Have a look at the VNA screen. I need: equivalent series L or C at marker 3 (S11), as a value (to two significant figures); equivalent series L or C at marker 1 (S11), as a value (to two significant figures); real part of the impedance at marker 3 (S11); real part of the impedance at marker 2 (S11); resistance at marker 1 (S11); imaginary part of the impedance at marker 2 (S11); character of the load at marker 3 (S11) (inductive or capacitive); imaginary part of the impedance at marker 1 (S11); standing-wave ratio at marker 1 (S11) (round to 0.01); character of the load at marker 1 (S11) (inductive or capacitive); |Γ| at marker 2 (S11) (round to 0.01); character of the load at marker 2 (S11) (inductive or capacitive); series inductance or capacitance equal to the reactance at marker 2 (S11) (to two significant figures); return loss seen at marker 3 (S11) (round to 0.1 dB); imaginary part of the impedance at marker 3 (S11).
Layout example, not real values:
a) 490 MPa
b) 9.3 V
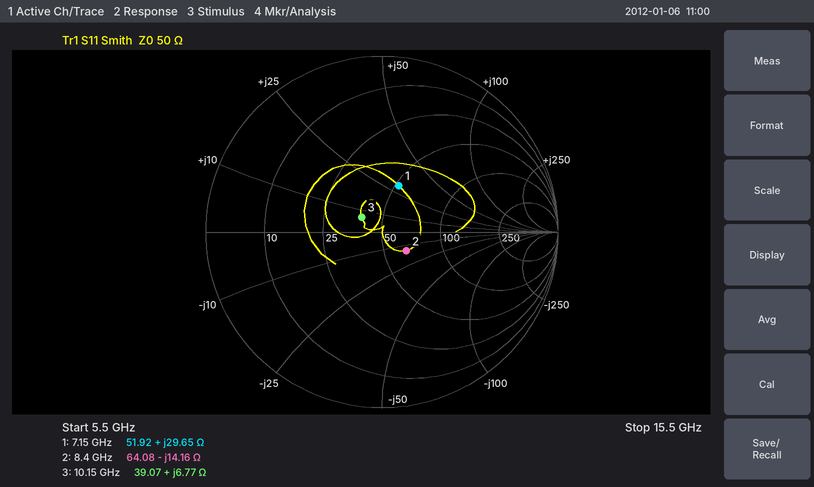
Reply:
a) 110 pH
b) 660 pH
c) 39.07 Ω
d) 64.08 Ω
e) 51.92 Ω
f) -14.16 Ω
g) inductive
h) +29.65 Ω
i) 1.78
j) inductive
k) 0.17
l) capacitive
m) 1.3 pF
n) 16.8 dB
o) +6.77 Ω
